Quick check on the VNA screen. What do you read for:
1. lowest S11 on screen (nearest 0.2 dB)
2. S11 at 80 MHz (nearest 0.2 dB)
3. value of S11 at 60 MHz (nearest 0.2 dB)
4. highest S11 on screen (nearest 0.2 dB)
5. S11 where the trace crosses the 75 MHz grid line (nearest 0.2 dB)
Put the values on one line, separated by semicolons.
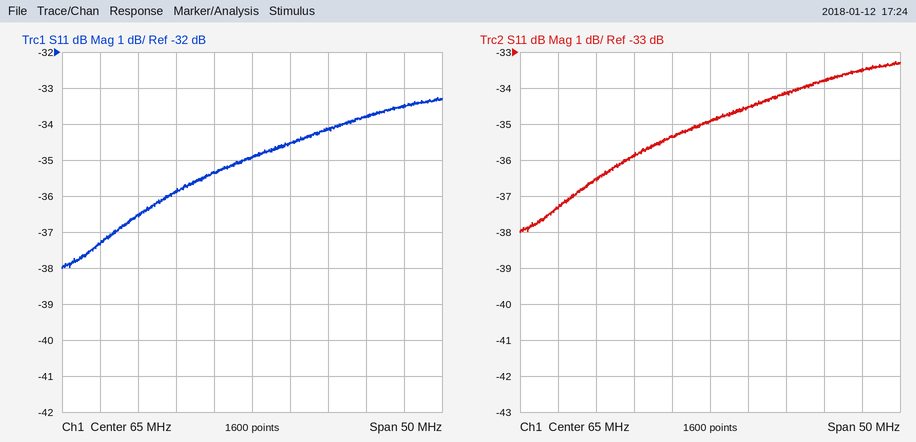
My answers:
-38.0 dB; -33.8 dB; -35.4 dB; -33.2 dB; -34.2 dB
